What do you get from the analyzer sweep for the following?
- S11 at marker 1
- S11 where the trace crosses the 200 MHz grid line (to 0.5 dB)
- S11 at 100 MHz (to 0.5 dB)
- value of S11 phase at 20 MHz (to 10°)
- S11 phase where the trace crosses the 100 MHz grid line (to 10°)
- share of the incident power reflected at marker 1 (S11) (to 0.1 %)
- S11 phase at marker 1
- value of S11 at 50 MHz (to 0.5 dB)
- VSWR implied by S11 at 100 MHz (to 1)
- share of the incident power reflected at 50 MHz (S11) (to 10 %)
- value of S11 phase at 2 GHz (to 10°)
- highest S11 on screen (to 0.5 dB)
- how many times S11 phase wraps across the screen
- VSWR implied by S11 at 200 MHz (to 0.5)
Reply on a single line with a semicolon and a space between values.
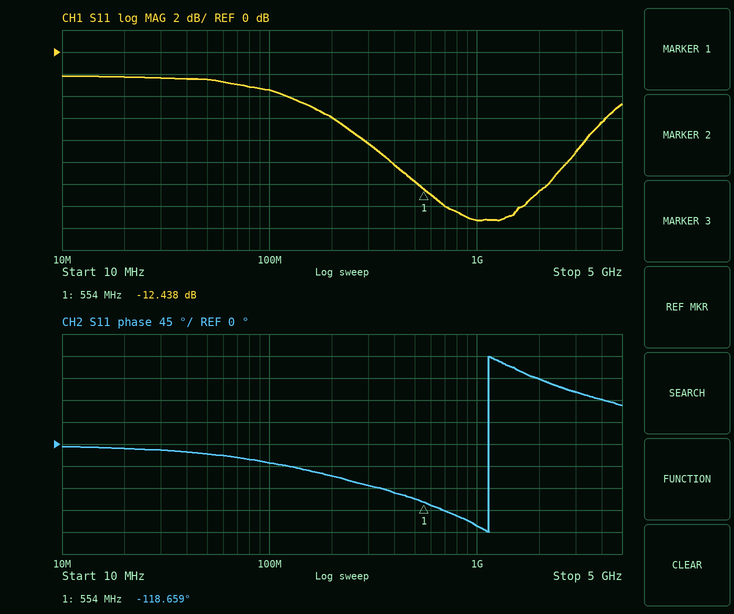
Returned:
-12.438 dB; -6.0 dB; -3.5 dB; -10°; -40°; 5.7 %; -118.659°; -2.5 dB; 5; 60 %; 130°; -2.0 dB; 1; 3.0
